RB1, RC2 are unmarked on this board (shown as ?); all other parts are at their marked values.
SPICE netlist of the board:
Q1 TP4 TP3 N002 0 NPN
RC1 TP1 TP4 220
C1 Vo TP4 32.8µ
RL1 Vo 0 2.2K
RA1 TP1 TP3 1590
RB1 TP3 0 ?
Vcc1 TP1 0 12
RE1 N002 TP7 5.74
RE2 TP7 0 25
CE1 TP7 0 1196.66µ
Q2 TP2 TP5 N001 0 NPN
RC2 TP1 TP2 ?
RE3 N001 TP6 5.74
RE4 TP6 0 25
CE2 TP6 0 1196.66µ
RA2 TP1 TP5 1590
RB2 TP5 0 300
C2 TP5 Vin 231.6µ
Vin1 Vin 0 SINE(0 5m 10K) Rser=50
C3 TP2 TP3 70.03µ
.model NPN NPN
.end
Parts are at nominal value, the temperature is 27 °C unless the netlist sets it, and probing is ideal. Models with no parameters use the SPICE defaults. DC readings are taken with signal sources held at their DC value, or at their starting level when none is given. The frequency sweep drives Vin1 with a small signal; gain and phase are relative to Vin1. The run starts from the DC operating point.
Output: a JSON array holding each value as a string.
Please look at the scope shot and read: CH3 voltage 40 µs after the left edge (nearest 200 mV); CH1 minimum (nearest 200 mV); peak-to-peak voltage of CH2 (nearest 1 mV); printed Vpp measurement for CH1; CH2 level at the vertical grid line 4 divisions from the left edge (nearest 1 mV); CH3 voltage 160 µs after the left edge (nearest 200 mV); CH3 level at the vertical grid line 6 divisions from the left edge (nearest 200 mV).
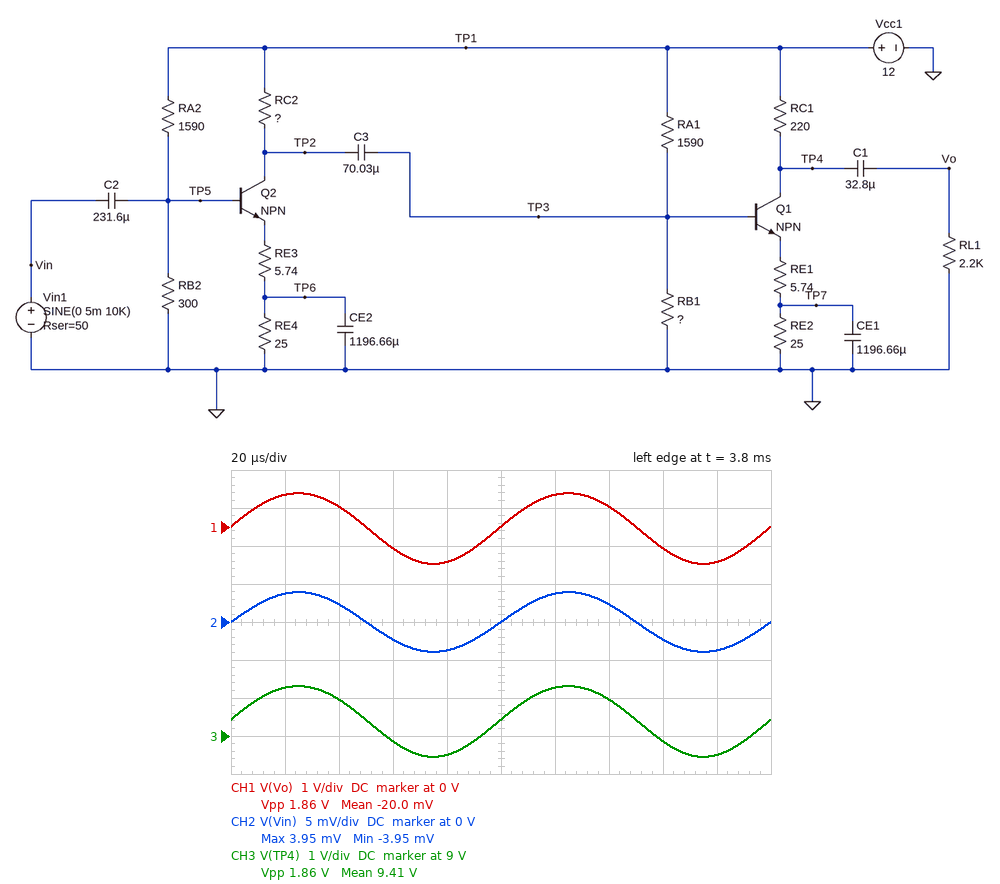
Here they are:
["10.0 V", "-1.0 V", "8 mV", "1.86 V", "-4 mV", "8.8 V", "10.2 V"]
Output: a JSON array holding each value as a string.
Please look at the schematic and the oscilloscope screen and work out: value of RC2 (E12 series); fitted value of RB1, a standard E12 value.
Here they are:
["120 Ω", "180 Ω"]
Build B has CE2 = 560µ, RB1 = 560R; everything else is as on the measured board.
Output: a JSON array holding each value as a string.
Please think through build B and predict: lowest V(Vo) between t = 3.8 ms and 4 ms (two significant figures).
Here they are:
["-5.2 mV"]
